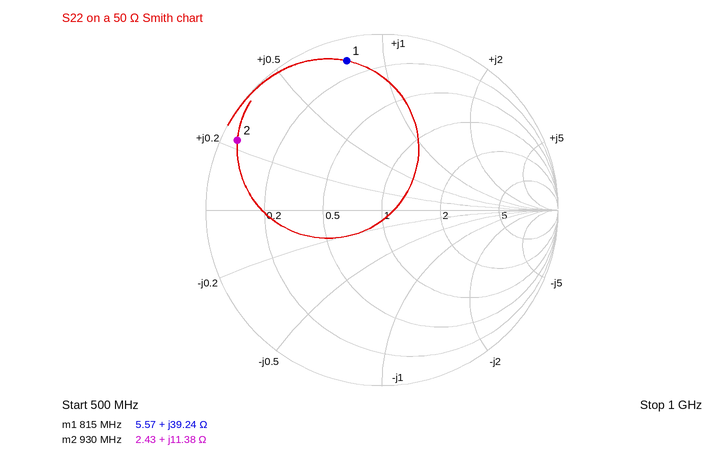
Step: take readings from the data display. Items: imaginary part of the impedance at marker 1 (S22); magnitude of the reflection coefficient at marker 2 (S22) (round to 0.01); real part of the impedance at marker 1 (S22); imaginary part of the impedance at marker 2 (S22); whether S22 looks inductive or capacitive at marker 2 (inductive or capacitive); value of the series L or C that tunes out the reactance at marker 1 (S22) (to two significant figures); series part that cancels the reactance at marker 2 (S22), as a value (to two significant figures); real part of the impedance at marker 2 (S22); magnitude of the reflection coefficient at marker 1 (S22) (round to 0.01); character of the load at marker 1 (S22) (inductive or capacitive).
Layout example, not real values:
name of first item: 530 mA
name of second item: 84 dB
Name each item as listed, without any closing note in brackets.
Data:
imaginary part of the impedance at marker 1: +39.24 Ω
magnitude of the reflection coefficient at marker 2 (S22): 0.91
real part of the impedance at marker 1: 5.57 Ω
imaginary part of the impedance at marker 2: +11.38 Ω
whether S22 looks inductive or capacitive at marker 2: inductive
value of the series L or C that tunes out the reactance at marker 1 (S22): 5.0 pF
series part that cancels the reactance at marker 2 (S22), as a value: 15 pF
real part of the impedance at marker 2: 2.43 Ω
magnitude of the reflection coefficient at marker 1 (S22): 0.87
character of the load at marker 1 (S22): inductive
